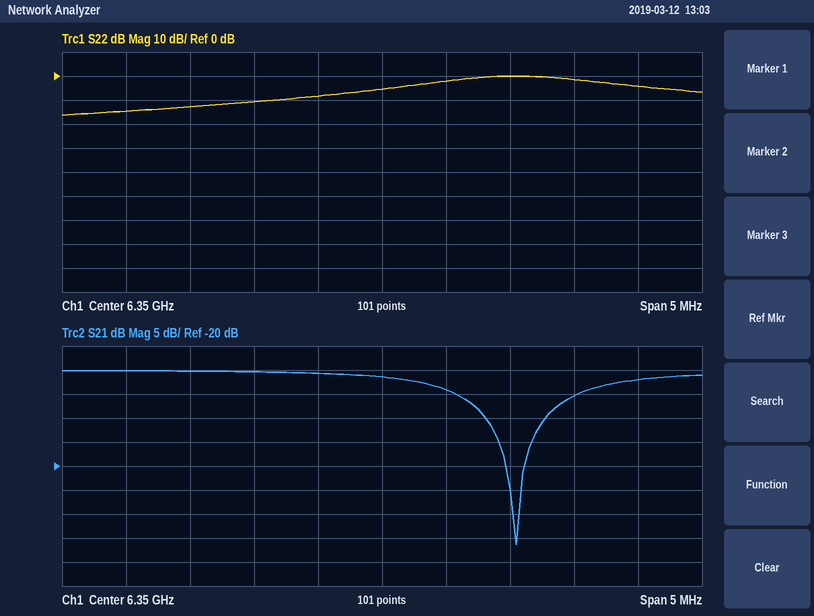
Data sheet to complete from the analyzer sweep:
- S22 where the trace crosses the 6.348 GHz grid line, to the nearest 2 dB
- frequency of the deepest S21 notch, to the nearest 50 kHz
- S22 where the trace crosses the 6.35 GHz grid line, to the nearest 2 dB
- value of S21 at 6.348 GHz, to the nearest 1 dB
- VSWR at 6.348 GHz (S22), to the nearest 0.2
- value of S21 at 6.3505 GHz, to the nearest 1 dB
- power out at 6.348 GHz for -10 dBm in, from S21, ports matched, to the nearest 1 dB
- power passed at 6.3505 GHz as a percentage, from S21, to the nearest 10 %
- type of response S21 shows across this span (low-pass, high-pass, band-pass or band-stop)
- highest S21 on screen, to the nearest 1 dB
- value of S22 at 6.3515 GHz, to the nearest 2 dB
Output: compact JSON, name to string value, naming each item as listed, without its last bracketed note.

{"S22 where the trace crosses the 6.348 GHz grid line, to the nearest 2 dB": "-14 dB", "frequency of the deepest S21 notch, to the nearest 50 kHz": "6.35105 GHz", "S22 where the trace crosses the 6.35 GHz grid line, to the nearest 2 dB": "-6 dB", "value of S21 at 6.348 GHz, to the nearest 1 dB": "0 dB", "VSWR at 6.348 GHz (S22), to the nearest 0.2": "1.4", "value of S21 at 6.3505 GHz, to the nearest 1 dB": "-4 dB", "power out at 6.348 GHz for -10 dBm in, from S21, ports matched, to the nearest 1 dB": "-10 dBm", "power passed at 6.3505 GHz as a percentage, from S21, to the nearest 10 %": "40 %", "type of response S21 shows across this span": "band-stop", "highest S21 on screen, to the nearest 1 dB": "0 dB", "value of S22 at 6.3515 GHz, to the nearest 2 dB": "-2 dB"}
